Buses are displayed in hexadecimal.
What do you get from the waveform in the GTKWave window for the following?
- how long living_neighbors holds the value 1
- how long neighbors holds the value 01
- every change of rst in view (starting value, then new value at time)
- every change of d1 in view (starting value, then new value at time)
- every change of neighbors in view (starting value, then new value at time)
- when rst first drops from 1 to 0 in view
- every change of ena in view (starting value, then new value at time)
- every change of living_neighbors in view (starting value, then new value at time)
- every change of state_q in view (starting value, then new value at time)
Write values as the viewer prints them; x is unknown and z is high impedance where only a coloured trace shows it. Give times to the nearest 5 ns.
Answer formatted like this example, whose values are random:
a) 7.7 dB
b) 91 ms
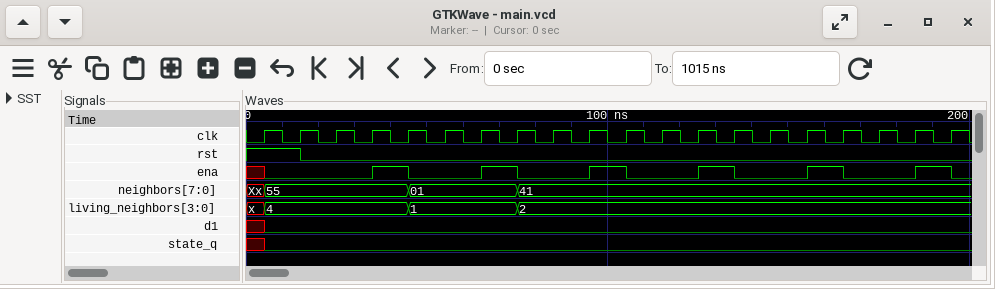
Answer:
a) 30 ns
b) 30 ns
c) 1, 0 at 15 ns
d) x, 0 at 5 ns
e) Xx, 55 at 5 ns, 01 at 45 ns, 41 at 75 ns
f) 15 ns
g) x, 0 at 5 ns, 1 at 35 ns, 0 at 45 ns, 1 at 65 ns, 0 at 75 ns, 1 at 95 ns, 0 at 105 ns, 1 at 125 ns, 0 at 135 ns, 1 at 155 ns, 0 at 165 ns, 1 at 185 ns, 0 at 195 ns
h) x, 4 at 5 ns, 1 at 45 ns, 2 at 75 ns
i) x, 0 at 5 ns
